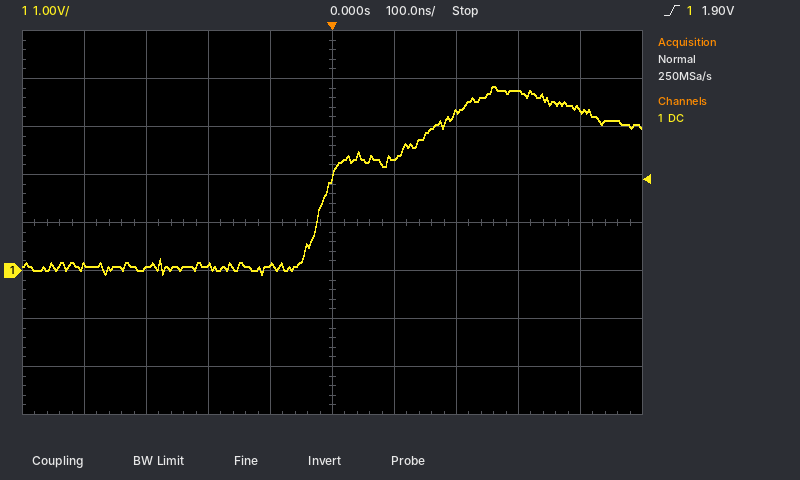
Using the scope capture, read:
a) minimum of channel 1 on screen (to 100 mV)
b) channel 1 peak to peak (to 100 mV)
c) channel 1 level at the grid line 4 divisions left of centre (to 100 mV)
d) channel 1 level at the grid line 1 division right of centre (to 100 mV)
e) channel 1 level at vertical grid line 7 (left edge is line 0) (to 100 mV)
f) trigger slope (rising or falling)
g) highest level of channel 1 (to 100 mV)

-100 mV
3.9 V
100 mV
2.3 V
3.3 V
rising
3.8 V
